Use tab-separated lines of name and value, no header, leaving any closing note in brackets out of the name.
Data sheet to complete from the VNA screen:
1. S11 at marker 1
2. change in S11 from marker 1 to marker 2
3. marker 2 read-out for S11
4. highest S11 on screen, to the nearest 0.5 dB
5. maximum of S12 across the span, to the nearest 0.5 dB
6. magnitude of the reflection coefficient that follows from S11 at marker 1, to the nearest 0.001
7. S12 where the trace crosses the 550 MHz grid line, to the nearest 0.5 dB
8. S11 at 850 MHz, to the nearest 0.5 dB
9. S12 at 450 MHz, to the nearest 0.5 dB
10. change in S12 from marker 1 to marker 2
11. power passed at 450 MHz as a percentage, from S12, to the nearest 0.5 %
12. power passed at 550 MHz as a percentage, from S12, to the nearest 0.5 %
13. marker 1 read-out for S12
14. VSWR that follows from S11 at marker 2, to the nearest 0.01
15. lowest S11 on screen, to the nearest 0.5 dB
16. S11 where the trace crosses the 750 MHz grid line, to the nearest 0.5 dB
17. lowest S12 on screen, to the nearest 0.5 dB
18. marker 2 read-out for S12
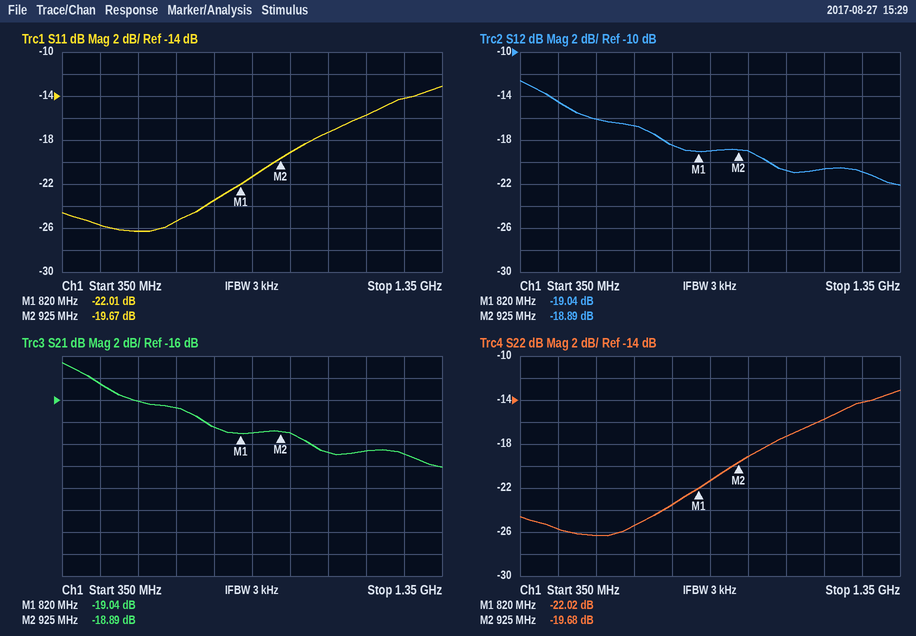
S11 at marker 1	-22.01 dB
change in S11 from marker 1 to marker 2	2.34 dB
marker 2 read-out for S11	-19.67 dB
highest S11 on screen, to the nearest 0.5 dB	-13.0 dB
maximum of S12 across the span, to the nearest 0.5 dB	-12.5 dB
magnitude of the reflection coefficient that follows from S11 at marker 1, to the nearest 0.001	0.079
S12 where the trace crosses the 550 MHz grid line, to the nearest 0.5 dB	-16.0 dB
S11 at 850 MHz, to the nearest 0.5 dB	-21.5 dB
S12 at 450 MHz, to the nearest 0.5 dB	-14.5 dB
change in S12 from marker 1 to marker 2	0.15 dB
power passed at 450 MHz as a percentage, from S12, to the nearest 0.5 %	3.5 %
power passed at 550 MHz as a percentage, from S12, to the nearest 0.5 %	2.5 %
marker 1 read-out for S12	-19.04 dB
VSWR that follows from S11 at marker 2, to the nearest 0.01	1.23
lowest S11 on screen, to the nearest 0.5 dB	-26.5 dB
S11 where the trace crosses the 750 MHz grid line, to the nearest 0.5 dB	-23.5 dB
lowest S12 on screen, to the nearest 0.5 dB	-22.0 dB
marker 2 read-out for S12	-18.89 dB
